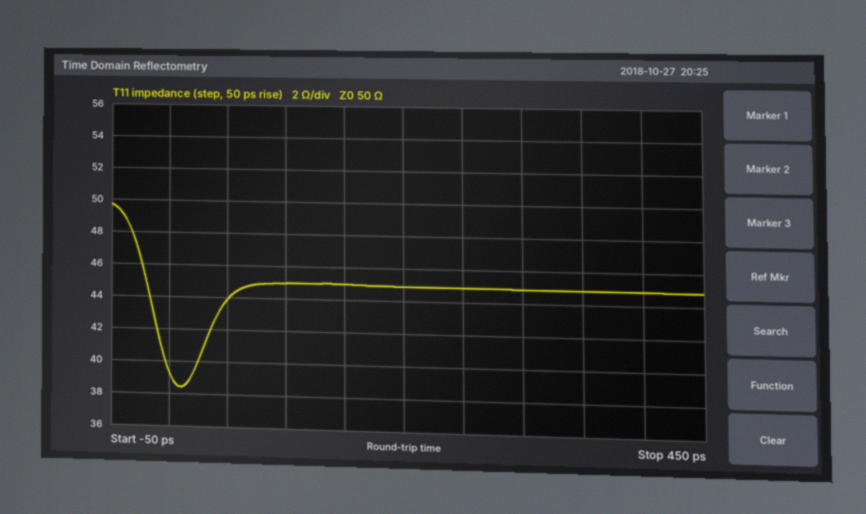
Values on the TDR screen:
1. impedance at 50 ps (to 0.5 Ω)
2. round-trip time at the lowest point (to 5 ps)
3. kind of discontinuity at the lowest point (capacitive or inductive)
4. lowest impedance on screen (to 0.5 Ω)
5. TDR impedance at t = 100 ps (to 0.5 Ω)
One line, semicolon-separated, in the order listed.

44.0 Ω; 10 ps; capacitive; 38.5 Ω; 45.0 Ω
